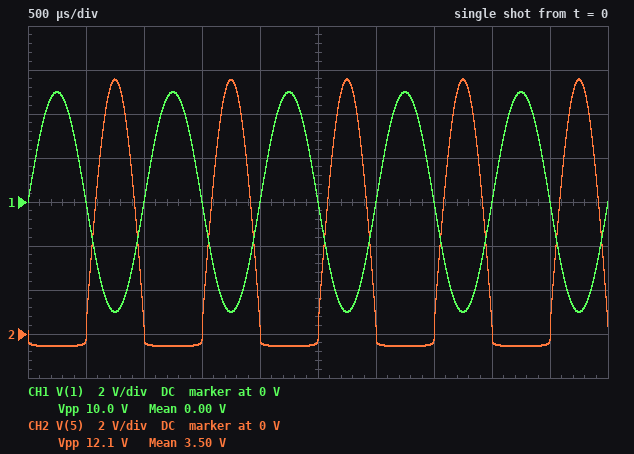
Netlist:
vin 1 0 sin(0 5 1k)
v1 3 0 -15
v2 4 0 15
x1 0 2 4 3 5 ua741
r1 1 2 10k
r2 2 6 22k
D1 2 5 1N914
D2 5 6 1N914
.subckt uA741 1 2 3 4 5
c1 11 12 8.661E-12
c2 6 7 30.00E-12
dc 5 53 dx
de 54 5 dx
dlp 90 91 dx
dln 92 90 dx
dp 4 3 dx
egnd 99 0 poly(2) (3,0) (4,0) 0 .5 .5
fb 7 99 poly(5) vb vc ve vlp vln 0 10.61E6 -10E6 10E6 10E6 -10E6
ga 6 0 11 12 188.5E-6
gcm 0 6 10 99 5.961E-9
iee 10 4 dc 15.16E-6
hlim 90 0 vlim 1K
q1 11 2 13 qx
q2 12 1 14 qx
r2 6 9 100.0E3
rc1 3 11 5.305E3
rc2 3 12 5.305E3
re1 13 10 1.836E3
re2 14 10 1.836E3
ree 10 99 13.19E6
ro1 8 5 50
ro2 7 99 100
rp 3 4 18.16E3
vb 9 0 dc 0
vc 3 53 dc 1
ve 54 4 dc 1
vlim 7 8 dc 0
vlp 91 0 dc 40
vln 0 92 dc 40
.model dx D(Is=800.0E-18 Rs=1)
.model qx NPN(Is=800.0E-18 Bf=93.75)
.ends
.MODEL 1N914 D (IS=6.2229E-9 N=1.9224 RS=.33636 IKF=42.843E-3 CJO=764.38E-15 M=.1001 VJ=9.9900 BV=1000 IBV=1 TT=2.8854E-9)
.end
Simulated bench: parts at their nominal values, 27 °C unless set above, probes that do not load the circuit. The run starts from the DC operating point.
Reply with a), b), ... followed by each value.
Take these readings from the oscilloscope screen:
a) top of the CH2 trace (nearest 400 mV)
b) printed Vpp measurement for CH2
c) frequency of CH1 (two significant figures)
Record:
a) 11.6 V
b) 12.1 V
c) 1.0 kHz
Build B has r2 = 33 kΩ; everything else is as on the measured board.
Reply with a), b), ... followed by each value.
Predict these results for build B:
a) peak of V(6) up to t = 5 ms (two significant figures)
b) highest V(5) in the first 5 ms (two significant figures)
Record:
a) 14 V
b) 15 V
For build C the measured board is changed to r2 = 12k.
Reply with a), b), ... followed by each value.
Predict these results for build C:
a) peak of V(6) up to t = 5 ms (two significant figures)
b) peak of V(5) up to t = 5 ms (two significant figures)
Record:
a) 6.0 V
b) 6.6 V
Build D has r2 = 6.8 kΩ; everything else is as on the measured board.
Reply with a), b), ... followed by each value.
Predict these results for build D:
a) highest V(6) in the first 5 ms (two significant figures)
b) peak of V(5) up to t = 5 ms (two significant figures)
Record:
a) 3.4 V
b) 4.0 V
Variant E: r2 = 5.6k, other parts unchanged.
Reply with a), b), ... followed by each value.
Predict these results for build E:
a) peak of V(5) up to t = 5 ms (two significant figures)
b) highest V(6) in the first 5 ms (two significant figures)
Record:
a) 3.4 V
b) 2.8 V
